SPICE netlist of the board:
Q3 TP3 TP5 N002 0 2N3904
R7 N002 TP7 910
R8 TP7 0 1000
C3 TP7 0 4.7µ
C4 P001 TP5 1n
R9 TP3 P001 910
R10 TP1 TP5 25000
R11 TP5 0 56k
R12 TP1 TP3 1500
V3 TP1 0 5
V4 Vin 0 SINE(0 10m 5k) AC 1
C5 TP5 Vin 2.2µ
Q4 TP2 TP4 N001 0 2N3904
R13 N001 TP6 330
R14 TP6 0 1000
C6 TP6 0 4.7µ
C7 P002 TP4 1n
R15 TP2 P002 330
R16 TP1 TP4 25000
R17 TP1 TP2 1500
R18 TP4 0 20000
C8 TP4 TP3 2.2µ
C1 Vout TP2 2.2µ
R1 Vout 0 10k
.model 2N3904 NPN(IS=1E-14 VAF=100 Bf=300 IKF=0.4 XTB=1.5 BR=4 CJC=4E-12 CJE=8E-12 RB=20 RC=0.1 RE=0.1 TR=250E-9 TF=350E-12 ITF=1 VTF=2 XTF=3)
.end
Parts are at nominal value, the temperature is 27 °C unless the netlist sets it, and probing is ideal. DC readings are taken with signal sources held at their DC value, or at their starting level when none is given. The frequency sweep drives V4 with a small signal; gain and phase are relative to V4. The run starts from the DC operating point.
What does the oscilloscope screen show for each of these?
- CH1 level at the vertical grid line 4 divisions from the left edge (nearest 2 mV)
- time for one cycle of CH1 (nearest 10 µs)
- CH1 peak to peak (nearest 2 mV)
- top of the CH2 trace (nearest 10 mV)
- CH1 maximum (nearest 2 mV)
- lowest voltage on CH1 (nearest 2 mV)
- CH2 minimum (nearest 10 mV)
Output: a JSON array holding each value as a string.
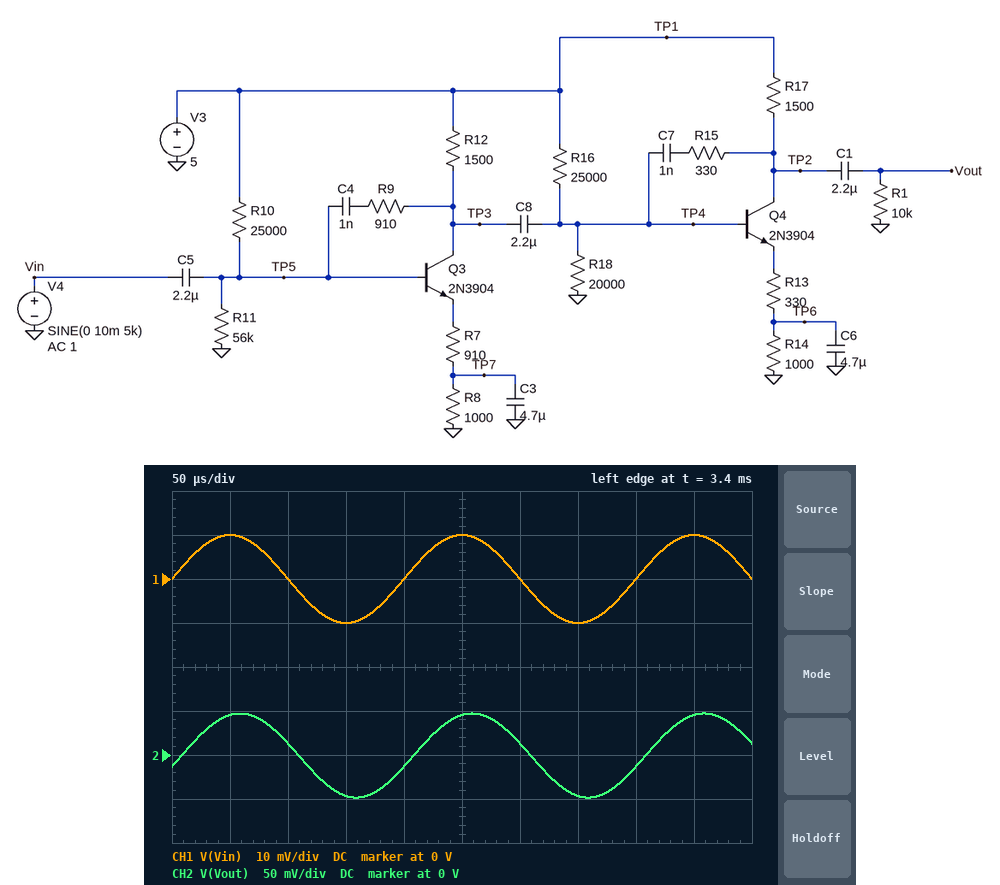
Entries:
["0 V", "200 µs", "20 mV", "50 mV", "10 mV", "-10 mV", "-50 mV"]
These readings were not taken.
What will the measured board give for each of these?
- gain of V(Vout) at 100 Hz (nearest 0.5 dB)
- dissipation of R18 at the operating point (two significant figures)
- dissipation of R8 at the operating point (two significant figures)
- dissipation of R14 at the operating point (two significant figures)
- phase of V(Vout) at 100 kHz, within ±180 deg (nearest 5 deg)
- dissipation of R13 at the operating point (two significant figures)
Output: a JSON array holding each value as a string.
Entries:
["9.0 dB", "240 µW", "2.0 mW", "1.3 mW", "-115 deg", "430 µW"]
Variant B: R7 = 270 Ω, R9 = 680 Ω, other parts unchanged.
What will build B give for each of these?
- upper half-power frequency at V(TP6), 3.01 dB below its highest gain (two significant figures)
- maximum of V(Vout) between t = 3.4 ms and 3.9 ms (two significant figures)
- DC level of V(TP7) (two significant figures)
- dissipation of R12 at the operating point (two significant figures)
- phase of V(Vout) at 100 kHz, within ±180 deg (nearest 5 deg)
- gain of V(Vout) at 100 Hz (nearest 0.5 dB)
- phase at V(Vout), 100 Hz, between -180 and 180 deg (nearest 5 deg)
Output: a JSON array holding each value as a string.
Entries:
["470 Hz", "41 mV", "1.8 V", "4.7 mW", "-110 deg", "0.5 dB", "135 deg"]
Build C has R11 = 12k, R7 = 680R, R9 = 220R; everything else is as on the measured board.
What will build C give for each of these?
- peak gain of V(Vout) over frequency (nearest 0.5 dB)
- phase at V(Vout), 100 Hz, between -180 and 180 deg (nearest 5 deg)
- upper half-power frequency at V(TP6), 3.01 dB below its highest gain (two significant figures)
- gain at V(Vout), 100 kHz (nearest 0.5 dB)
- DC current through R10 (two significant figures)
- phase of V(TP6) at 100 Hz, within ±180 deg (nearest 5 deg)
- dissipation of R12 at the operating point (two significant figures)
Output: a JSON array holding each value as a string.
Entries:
["16.5 dB", "65 deg", "240 Hz", "1.5 dB", "140 µA", "170 deg", "490 µW"]
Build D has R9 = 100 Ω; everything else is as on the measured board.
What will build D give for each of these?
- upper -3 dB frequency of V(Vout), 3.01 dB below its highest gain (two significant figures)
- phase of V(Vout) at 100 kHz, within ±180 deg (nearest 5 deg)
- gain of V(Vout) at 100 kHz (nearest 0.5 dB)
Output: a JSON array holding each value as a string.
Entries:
["19 kHz", "-120 deg", "0 dB"]
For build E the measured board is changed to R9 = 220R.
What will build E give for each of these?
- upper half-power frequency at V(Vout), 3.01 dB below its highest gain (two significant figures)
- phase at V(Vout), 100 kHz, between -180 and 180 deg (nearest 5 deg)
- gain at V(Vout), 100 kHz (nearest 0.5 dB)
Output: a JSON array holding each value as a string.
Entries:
["19 kHz", "-120 deg", "-0.5 dB"]
